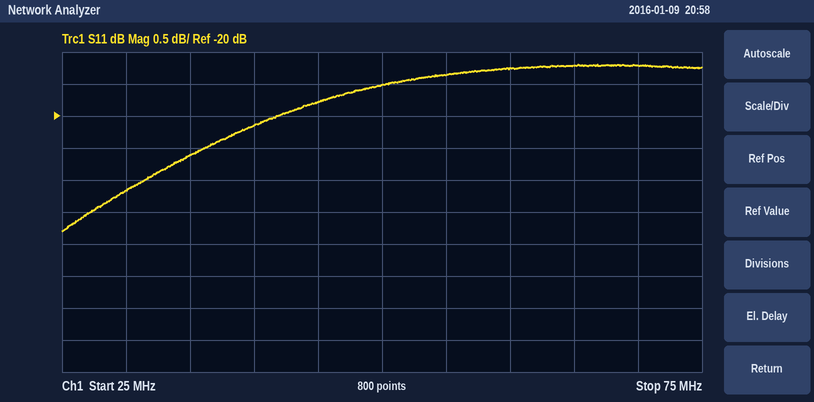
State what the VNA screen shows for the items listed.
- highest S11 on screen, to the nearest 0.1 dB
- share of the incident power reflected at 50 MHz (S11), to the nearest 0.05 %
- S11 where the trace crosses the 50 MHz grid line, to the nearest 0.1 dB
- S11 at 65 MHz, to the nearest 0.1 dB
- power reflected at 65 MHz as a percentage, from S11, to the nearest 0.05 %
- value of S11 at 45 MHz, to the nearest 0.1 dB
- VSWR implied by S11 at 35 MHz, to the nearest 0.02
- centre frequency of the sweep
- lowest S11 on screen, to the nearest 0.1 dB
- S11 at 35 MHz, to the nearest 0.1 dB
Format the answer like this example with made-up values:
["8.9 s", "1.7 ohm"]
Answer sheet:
["-19.2 dB", "1.10 %", "-19.5 dB", "-19.2 dB", "1.20 %", "-19.8 dB", "1.20", "50 MHz", "-21.8 dB", "-20.6 dB"]
